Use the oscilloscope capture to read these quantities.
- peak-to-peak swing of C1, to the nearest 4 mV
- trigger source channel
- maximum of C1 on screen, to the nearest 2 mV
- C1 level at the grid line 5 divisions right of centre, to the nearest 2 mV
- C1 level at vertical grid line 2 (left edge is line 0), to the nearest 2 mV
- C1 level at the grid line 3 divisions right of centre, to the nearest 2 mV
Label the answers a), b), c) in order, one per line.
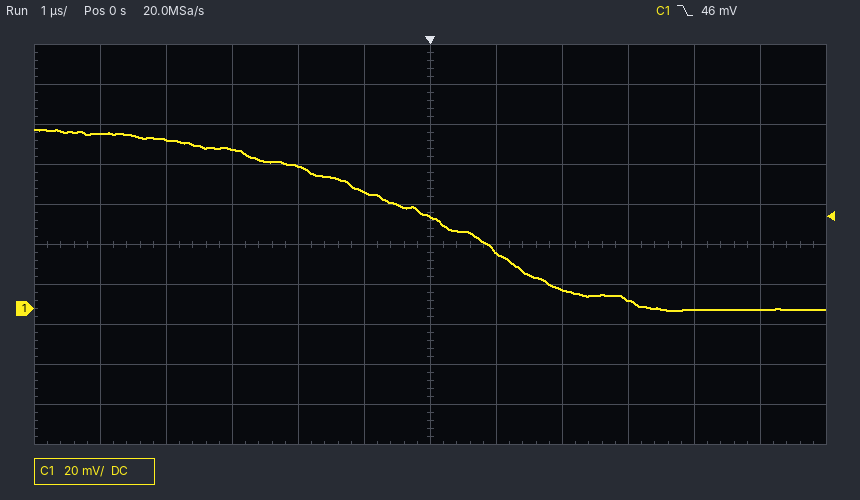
a) 92 mV
b) C1
c) 90 mV
d) 0 mV
e) 84 mV
f) 4 mV
